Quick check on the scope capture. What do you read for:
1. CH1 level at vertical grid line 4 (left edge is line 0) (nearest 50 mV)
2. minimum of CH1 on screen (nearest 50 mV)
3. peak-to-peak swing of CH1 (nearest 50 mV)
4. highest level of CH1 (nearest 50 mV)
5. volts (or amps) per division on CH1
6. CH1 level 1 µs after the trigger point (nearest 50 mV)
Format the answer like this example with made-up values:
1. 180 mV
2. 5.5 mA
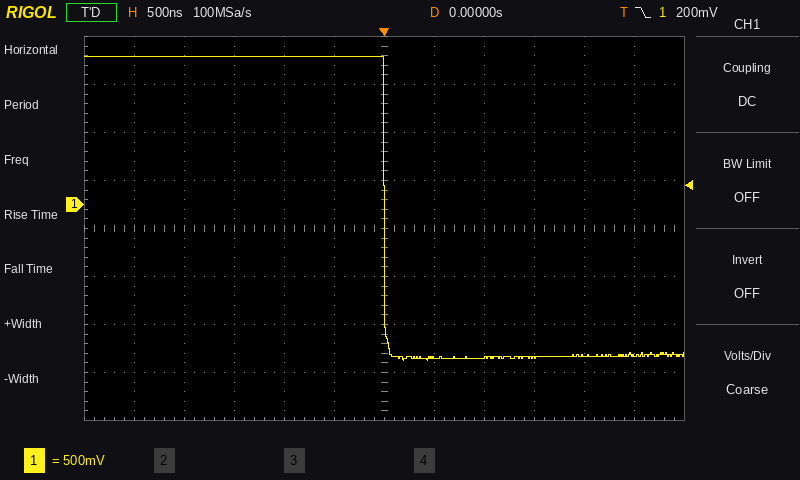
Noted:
1. 1.55 V
2. -1.60 V
3. 3.15 V
4. 1.55 V
5. 500 mV
6. -1.60 V
